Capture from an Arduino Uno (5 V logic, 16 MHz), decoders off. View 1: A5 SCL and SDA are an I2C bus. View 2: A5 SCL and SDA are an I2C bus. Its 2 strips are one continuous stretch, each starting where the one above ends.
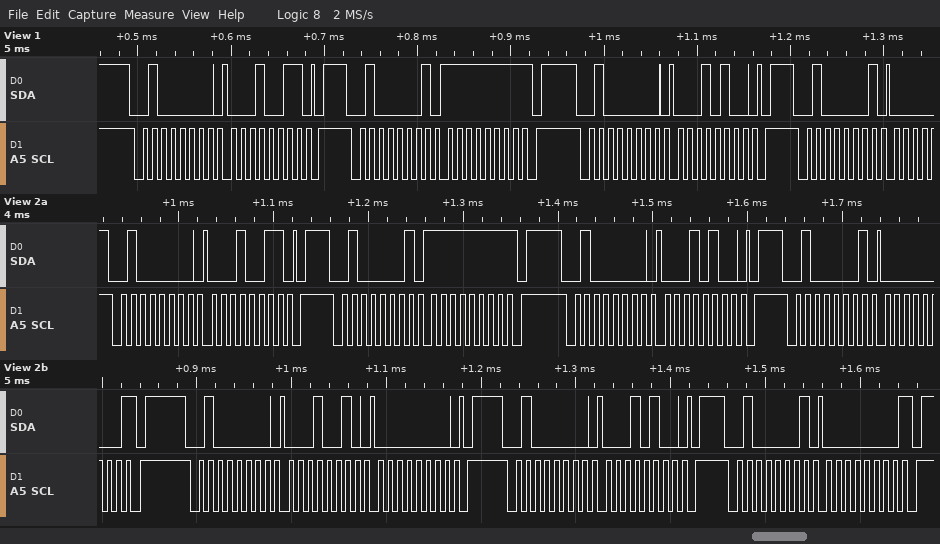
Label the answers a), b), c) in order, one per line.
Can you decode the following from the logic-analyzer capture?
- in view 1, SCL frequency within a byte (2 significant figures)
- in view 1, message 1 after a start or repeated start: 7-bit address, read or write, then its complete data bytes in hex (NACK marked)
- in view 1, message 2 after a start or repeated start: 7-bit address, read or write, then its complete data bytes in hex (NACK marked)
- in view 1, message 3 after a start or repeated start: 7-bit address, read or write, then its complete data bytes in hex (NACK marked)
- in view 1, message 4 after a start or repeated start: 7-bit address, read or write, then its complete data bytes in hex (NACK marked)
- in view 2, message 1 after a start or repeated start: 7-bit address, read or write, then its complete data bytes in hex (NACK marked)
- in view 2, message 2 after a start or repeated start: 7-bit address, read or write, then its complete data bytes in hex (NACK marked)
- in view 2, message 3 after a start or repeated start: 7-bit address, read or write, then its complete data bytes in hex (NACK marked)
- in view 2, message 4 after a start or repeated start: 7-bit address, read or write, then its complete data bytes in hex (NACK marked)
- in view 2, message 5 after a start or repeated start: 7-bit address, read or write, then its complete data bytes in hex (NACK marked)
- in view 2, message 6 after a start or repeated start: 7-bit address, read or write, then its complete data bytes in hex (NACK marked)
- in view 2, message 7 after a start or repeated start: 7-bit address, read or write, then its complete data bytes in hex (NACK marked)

a) 100 kHz
b) 0x20 write: 13
c) 0x20 read: FF NACK
d) 0x20 write: 14
e) 0x20 read
f) 0x20 write: 13
g) 0x20 read: FF NACK
h) 0x20 write: 14
i) 0x20 read: 00 NACK
j) 0x20 write: 12 00
k) 0x20 write: 14
l) 0x20 read: 00 NACK
